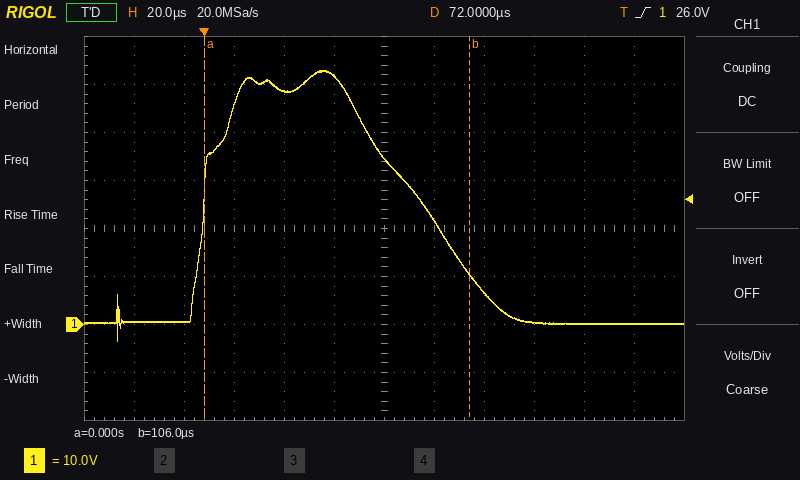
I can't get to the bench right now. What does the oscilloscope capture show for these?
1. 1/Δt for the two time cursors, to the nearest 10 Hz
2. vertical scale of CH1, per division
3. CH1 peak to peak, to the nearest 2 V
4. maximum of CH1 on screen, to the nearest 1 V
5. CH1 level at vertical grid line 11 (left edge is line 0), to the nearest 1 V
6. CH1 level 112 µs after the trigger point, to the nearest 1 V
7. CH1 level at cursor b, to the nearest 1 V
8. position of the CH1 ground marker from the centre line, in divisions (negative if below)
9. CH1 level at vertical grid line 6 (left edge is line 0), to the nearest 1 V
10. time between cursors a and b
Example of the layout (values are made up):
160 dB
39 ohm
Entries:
9.43 kHz
10 V
56 V
53 V
0 V
7 V
10 V
-2.0 div
35 V
106 µs
